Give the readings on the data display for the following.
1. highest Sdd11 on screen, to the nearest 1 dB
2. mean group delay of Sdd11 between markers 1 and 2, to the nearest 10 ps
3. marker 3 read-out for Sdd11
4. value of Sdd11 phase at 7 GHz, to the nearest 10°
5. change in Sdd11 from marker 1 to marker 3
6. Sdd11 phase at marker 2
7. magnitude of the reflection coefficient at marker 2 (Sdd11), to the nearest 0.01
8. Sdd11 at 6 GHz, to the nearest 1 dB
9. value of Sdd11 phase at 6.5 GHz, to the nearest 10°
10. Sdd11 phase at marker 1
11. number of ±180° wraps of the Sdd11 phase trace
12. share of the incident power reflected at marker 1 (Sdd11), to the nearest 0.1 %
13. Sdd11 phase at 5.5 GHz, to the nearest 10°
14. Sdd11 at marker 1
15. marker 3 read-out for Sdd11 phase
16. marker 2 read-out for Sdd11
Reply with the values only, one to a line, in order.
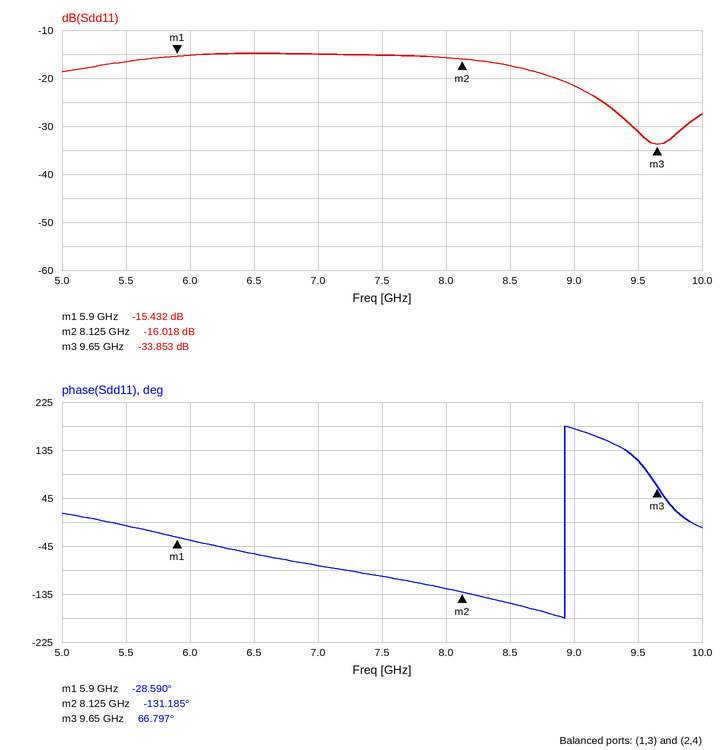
-15 dB
130 ps
-33.853 dB
-80°
-18.421 dB
-131.185°
0.16
-15 dB
-60°
-28.590°
1
2.9 %
-10°
-15.432 dB
66.797°
-16.018 dB
